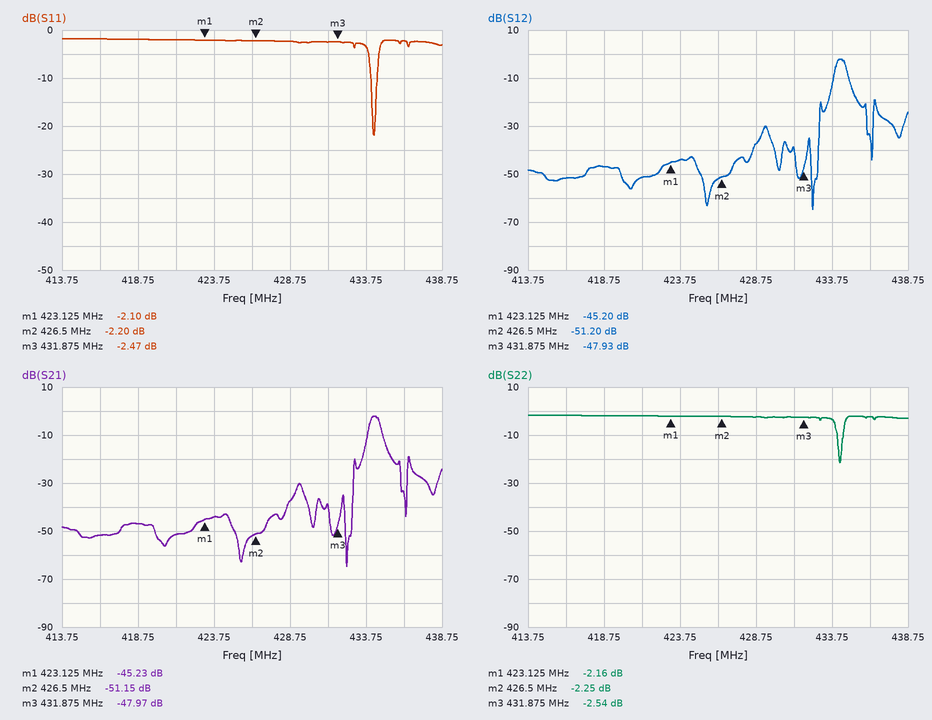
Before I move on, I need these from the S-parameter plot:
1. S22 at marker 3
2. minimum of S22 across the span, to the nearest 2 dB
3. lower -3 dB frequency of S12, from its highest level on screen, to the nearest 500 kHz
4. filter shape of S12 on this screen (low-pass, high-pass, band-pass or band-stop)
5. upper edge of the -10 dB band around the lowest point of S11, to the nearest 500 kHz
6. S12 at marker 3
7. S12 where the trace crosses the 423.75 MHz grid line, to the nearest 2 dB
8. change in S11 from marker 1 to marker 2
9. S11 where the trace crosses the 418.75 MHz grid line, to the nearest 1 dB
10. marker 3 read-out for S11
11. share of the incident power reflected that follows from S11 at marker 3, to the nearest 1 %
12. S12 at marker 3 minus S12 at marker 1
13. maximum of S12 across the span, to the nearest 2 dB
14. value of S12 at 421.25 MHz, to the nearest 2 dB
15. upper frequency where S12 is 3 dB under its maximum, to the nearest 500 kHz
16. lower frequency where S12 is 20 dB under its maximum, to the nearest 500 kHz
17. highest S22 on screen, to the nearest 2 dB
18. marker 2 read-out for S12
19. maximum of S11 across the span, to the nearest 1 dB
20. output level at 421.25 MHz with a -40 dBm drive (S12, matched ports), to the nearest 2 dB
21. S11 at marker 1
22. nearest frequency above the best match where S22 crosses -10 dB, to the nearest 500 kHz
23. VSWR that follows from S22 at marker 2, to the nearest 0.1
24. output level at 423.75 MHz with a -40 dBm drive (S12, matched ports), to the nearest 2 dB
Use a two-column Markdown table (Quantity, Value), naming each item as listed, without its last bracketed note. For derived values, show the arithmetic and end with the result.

| Quantity | Value |
|---|---|
| S22 at marker 3 | -2.54 dB |
| minimum of S22 across the span, to the nearest 2 dB | -22 dB |
| lower -3 dB frequency of S12, from its highest level on screen, to the nearest 500 kHz | 434.0 MHz |
| filter shape of S12 on this screen | band-pass |
| upper edge of the -10 dB band around the lowest point of S11, to the nearest 500 kHz | 434.5 MHz |
| S12 at marker 3 | -47.93 dB |
| S12 where the trace crosses the 423.75 MHz grid line, to the nearest 2 dB | -44 dB |
| change in S11 from marker 1 to marker 2 | -2.2 − (-2.1) = -0.10 dB |
| S11 where the trace crosses the 418.75 MHz grid line, to the nearest 1 dB | -2 dB |
| marker 3 read-out for S11 | -2.47 dB |
| share of the incident power reflected that follows from S11 at marker 3, to the nearest 1 % | 10^(-2.47/10) ≈ 57 % |
| S12 at marker 3 minus S12 at marker 1 | -47.93 − (-45.2) = -2.73 dB |
| maximum of S12 across the span, to the nearest 2 dB | -2 dB |
| value of S12 at 421.25 MHz, to the nearest 2 dB | -52 dB |
| upper frequency where S12 is 3 dB under its maximum, to the nearest 500 kHz | 434.5 MHz |
| lower frequency where S12 is 20 dB under its maximum, to the nearest 500 kHz | 433.5 MHz |
| highest S22 on screen, to the nearest 2 dB | -2 dB |
| marker 2 read-out for S12 | -51.20 dB |
| maximum of S11 across the span, to the nearest 1 dB | -2 dB |
| output level at 421.25 MHz with a -40 dBm drive (S12, matched ports), to the nearest 2 dB | -40 dBm + (-52 dB) = -92 dBm |
| S11 at marker 1 | -2.10 dB |
| nearest frequency above the best match where S22 crosses -10 dB, to the nearest 500 kHz | 434.5 MHz |
| VSWR that follows from S22 at marker 2, to the nearest 0.1 | (1 + 0.7718)/(1 − 0.7718) ≈ 7.8 |
| output level at 423.75 MHz with a -40 dBm drive (S12, matched ports), to the nearest 2 dB | -40 dBm + (-44 dB) = -84 dBm |
